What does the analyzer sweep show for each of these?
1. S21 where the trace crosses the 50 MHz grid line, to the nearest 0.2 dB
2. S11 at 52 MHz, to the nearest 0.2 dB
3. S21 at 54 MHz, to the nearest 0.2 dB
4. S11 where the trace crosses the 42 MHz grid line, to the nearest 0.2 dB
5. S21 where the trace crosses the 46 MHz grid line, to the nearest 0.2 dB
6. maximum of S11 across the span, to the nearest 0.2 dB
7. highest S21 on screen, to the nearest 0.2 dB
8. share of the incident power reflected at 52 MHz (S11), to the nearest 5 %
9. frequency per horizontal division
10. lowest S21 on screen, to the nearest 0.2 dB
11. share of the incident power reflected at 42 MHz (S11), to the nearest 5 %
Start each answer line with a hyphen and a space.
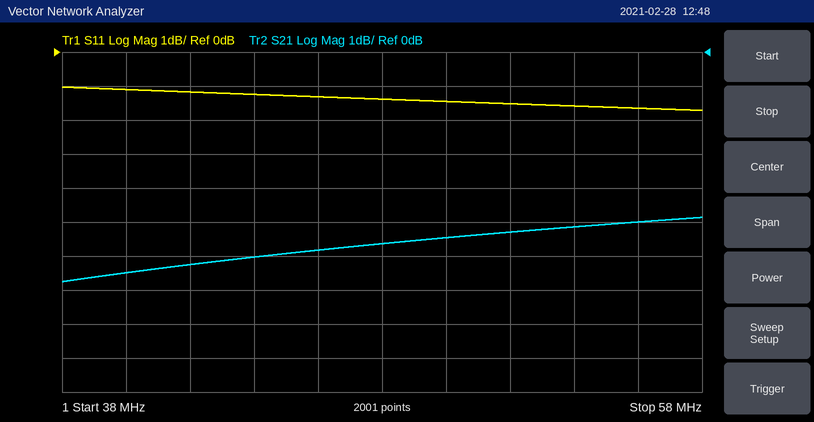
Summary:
- -5.4 dB
- -1.6 dB
- -5.2 dB
- -1.2 dB
- -5.8 dB
- -1.0 dB
- -4.8 dB
- 70 %
- 2 MHz
- -6.8 dB
- 75 %
